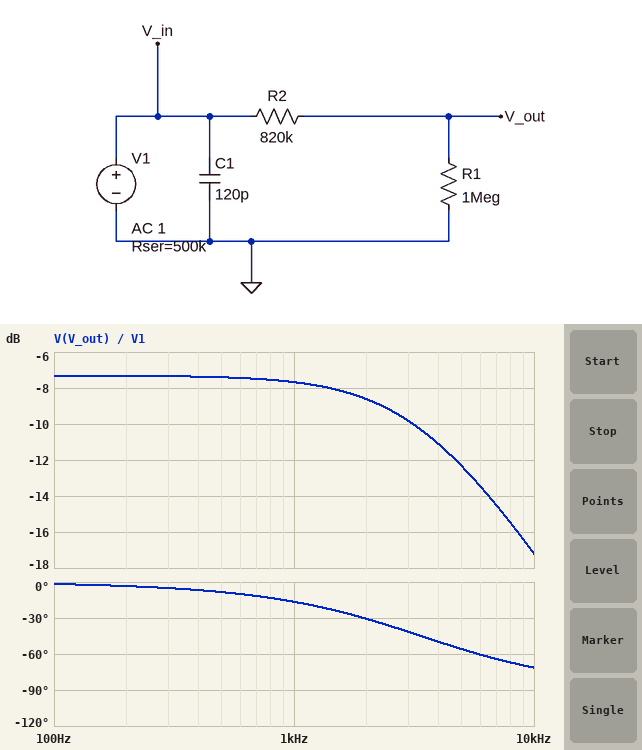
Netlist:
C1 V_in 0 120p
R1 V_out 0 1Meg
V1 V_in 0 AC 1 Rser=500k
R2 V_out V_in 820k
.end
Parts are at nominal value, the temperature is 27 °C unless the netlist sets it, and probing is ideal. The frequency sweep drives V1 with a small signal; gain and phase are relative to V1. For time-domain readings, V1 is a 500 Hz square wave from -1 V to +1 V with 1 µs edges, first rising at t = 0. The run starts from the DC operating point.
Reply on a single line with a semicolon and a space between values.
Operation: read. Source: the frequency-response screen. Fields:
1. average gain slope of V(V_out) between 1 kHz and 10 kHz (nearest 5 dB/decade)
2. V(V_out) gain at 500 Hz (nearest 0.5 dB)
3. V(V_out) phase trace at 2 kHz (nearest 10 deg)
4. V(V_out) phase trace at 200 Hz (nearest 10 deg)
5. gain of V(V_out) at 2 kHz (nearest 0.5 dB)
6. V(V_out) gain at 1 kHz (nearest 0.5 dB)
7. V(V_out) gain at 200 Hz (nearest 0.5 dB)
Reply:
-10 dB/decade; -7.5 dB; -30 deg; 0 deg; -8.5 dB; -7.5 dB; -7.5 dB
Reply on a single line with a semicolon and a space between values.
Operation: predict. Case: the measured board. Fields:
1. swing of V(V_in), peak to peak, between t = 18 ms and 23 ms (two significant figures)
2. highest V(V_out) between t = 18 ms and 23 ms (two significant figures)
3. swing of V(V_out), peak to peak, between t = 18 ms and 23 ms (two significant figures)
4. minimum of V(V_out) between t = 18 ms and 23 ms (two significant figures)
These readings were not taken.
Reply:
1.6 V; 430 mV; 860 mV; -430 mV
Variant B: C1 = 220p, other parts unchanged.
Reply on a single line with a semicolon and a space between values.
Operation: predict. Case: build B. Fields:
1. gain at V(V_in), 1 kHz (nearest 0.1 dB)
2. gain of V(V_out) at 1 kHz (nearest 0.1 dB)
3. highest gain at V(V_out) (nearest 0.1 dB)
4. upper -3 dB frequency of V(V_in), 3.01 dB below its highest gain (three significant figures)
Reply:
-3.2 dB; -8.4 dB; -7.3 dB; 1.84 kHz
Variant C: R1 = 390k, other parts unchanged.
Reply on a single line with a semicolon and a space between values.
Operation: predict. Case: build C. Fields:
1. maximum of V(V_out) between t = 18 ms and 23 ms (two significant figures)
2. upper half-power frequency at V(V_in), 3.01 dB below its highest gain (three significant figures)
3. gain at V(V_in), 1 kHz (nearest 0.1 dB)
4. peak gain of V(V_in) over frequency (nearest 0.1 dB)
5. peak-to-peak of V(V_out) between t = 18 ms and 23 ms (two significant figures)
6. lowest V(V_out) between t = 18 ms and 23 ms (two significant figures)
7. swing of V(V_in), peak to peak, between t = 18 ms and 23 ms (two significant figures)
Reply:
230 mV; 3.75 kHz; -3.3 dB; -3.0 dB; 460 mV; -230 mV; 1.4 V
